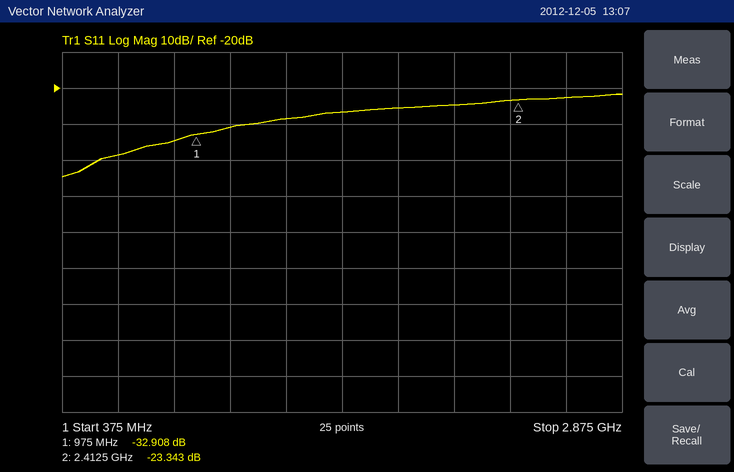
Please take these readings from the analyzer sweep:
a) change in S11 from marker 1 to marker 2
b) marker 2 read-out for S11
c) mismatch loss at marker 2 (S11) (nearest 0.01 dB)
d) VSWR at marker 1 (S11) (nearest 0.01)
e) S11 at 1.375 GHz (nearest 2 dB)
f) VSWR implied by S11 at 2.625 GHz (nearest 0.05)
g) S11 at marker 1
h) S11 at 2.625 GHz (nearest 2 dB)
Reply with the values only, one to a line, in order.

9.565 dB
-23.343 dB
0.02 dB
1.05
-28 dB
1.15
-32.908 dB
-22 dB
